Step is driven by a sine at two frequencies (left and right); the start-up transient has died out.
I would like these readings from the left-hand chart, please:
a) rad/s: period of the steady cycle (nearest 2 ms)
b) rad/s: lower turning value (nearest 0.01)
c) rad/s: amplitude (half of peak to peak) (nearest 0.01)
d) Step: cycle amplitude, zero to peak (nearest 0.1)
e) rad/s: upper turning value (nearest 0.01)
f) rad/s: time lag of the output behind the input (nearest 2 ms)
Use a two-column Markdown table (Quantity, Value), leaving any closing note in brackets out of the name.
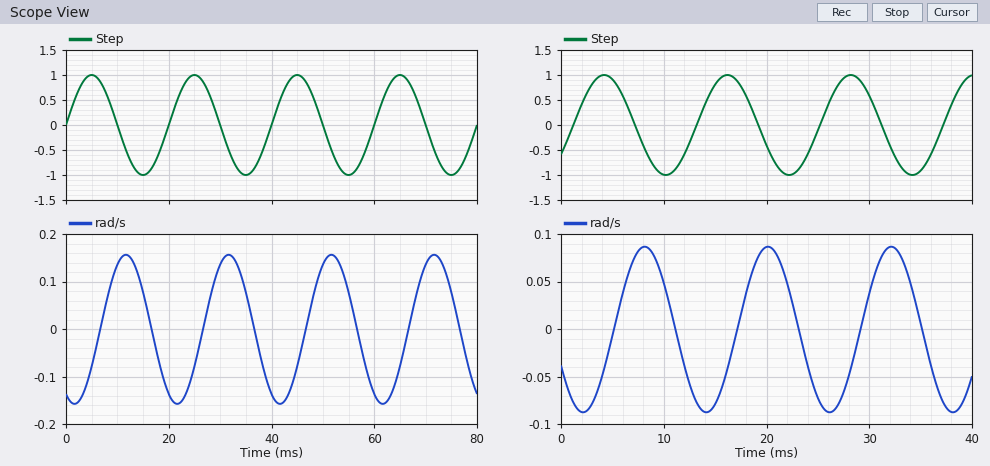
| Quantity | Value |
|---|---|
| rad/s: period of the steady cycle | 20 ms |
| rad/s: lower turning value | -0.16 |
| rad/s: amplitude (half of peak to peak) | 0.16 |
| Step: cycle amplitude, zero to peak | 1.0 |
| rad/s: upper turning value | 0.16 |
| rad/s: time lag of the output behind the input | 6 ms |
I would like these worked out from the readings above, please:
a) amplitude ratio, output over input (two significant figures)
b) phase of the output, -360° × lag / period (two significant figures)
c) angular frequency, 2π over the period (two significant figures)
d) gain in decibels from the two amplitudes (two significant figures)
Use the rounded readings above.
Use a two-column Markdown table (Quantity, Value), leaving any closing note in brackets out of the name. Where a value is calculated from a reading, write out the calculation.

| Quantity | Value |
|---|---|
| amplitude ratio, output over input | 0.16 / 1 = 0.16 |
| phase of the output, -360° × lag / period | -360 × 6 / 20 = -110° |
| angular frequency, 2π over the period | 2π / 20 = 0.31 rad/ms |
| gain in decibels from the two amplitudes | 20 log10(0.16 / 1) = -16 dB |
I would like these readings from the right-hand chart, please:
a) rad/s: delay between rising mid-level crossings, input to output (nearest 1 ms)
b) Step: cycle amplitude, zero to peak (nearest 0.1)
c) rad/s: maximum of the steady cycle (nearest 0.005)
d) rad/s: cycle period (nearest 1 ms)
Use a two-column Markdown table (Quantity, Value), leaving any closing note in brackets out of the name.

| Quantity | Value |
|---|---|
| rad/s: delay between rising mid-level crossings, input to output | 4 ms |
| Step: cycle amplitude, zero to peak | 1.0 |
| rad/s: maximum of the steady cycle | 0.085 |
| rad/s: cycle period | 12 ms |
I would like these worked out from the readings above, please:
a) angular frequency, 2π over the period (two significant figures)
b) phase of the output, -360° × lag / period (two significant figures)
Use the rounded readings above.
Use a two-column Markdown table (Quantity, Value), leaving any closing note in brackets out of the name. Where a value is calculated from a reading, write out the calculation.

| Quantity | Value |
|---|---|
| angular frequency, 2π over the period | 2π / 12 = 0.52 rad/ms |
| phase of the output, -360° × lag / period | -360 × 4 / 12 = -120° |
